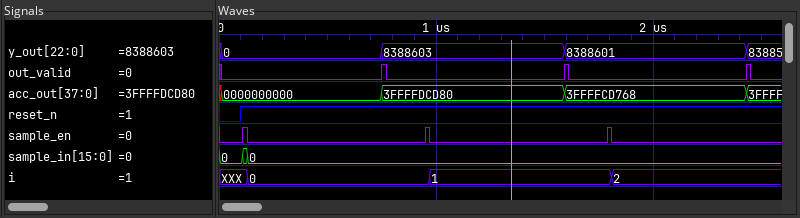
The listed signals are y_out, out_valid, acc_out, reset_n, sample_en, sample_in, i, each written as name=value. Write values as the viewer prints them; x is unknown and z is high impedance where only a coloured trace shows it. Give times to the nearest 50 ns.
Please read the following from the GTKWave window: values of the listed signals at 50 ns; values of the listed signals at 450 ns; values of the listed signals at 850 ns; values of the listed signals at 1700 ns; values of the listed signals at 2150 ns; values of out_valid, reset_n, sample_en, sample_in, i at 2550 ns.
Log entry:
y_out=0, out_valid=0, acc_out=0000000000, reset_n=0, sample_en=0, sample_in=0, i=XXX
y_out=0, out_valid=0, acc_out=0000000000, reset_n=1, sample_en=0, sample_in=0, i=0
y_out=8388603, out_valid=0, acc_out=3FFFFDCD80, reset_n=1, sample_en=0, sample_in=0, i=0
y_out=8388601, out_valid=0, acc_out=3FFFFCD768, reset_n=1, sample_en=0, sample_in=0, i=1
y_out=8388601, out_valid=0, acc_out=3FFFFCD768, reset_n=1, sample_en=0, sample_in=0, i=2
out_valid=0, reset_n=1, sample_en=0, sample_in=0, i=2
